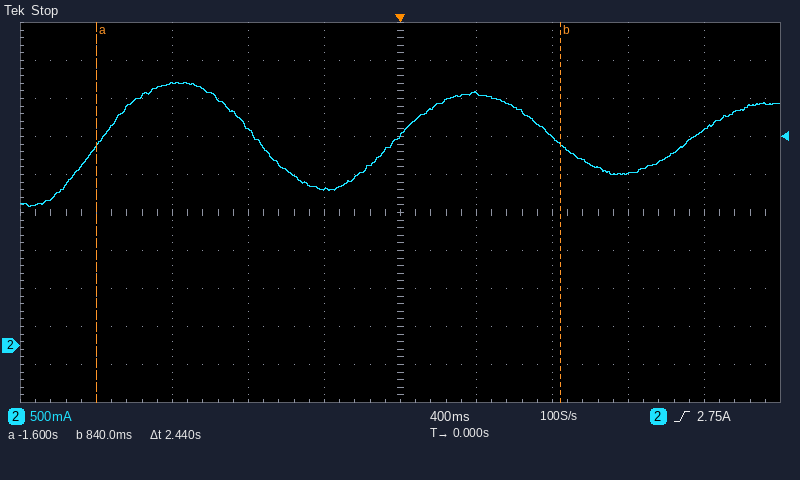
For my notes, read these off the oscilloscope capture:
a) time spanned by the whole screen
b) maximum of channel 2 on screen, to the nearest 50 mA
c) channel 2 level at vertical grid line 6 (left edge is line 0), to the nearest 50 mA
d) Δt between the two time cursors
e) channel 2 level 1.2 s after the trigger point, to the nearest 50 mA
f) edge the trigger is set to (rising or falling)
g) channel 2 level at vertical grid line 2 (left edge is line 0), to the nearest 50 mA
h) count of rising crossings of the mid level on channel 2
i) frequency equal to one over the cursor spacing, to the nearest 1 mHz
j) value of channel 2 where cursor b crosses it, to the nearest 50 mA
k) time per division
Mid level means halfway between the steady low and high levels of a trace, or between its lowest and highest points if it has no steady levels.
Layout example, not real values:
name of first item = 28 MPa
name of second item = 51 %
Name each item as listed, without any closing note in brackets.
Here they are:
time spanned by the whole screen = 4 s
maximum of channel 2 on screen, to the nearest 50 mA = 3.45 A
channel 2 level at vertical grid line 6 (left edge is line 0), to the nearest 50 mA = 3.30 A
Δt between the two time cursors = 2.44 s
channel 2 level 1.2 s after the trigger point, to the nearest 50 mA = 2.25 A
edge the trigger is set to = rising
channel 2 level at vertical grid line 2 (left edge is line 0), to the nearest 50 mA = 3.45 A
count of rising crossings of the mid level on channel 2 = 3
frequency equal to one over the cursor spacing, to the nearest 1 mHz = 410 mHz
value of channel 2 where cursor b crosses it, to the nearest 50 mA = 2.65 A
time per division = 400 ms
